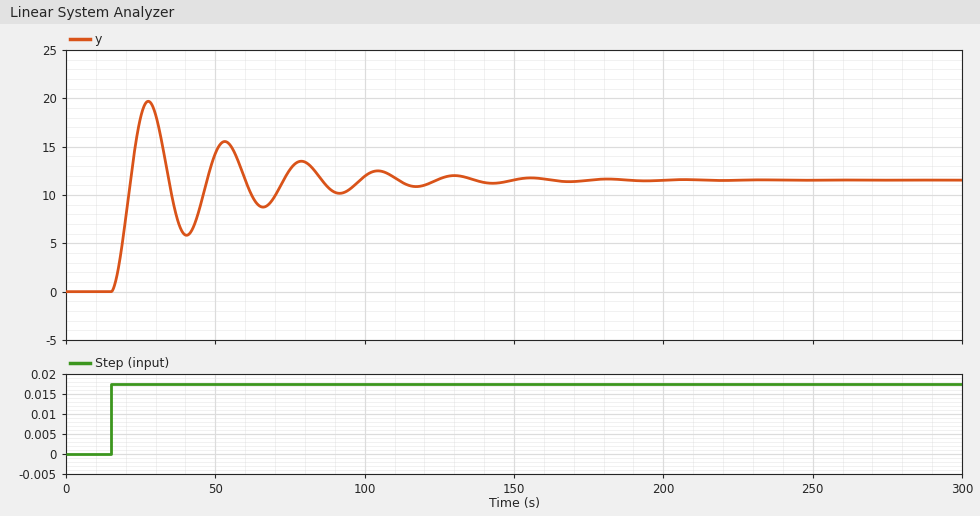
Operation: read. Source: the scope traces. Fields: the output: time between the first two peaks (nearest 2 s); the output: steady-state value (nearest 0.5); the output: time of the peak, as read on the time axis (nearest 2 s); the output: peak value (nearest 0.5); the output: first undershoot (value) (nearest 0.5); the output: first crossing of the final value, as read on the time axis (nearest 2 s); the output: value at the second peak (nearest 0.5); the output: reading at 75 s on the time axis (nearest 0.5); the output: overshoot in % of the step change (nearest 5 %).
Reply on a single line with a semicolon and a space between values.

26 s; 11.5; 28 s; 19.5; 6.0; 22 s; 15.5; 12.5; 70 %
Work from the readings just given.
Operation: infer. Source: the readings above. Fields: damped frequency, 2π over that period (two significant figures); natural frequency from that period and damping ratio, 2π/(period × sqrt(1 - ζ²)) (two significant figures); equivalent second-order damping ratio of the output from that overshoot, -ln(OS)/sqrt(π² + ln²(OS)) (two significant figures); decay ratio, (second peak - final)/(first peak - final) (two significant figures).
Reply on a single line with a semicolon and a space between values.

0.24 rad/s; 0.24 rad/s; 0.11; 0.50
